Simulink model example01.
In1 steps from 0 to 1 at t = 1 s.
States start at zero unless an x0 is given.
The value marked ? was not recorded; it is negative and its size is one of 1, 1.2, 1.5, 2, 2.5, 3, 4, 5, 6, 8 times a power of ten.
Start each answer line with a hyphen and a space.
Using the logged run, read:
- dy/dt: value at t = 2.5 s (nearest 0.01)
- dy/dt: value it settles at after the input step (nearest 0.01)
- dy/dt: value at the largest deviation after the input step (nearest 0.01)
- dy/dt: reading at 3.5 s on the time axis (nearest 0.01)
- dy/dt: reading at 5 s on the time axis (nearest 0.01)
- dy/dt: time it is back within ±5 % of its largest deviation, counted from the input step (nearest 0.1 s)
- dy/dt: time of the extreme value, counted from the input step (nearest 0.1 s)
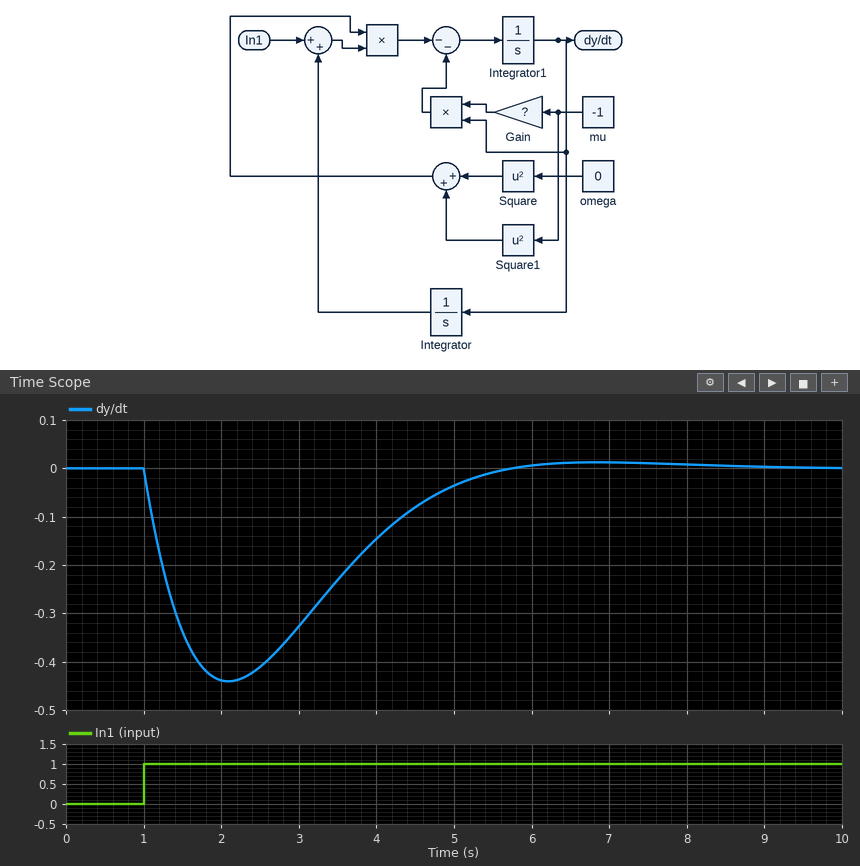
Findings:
- -0.41
- 0.00
- -0.44
- -0.23
- -0.04
- 4.2 s
- 1.1 s
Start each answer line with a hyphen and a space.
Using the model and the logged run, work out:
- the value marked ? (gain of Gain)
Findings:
- -1.5
